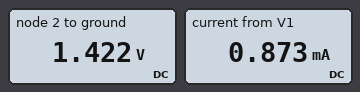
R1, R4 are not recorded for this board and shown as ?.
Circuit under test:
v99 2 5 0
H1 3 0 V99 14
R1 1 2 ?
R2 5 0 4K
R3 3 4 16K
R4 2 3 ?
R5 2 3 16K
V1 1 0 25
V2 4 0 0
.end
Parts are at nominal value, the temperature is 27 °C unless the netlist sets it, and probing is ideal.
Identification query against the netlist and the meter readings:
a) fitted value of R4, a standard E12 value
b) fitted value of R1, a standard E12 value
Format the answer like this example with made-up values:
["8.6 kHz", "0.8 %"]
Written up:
["3.3 kΩ", "27 kΩ"]
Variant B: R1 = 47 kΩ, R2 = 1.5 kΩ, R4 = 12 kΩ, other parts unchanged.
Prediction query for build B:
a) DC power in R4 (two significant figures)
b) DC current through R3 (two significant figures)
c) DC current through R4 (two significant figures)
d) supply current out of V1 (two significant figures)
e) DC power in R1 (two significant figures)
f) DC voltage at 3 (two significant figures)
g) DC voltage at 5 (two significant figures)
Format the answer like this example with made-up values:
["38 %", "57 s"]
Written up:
["33 µW", "370 nA", "53 µA", "520 µA", "13 mW", "6.0 mV", "640 mV"]
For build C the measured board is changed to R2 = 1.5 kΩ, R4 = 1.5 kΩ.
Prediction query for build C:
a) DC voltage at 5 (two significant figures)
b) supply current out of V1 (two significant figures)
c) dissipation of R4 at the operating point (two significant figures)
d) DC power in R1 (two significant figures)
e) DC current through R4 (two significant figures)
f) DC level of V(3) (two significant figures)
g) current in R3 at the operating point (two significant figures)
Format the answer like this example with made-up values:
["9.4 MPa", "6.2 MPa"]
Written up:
["650 mV", "900 µA", "280 µW", "22 mW", "430 µA", "6.1 mV", "380 nA"]
